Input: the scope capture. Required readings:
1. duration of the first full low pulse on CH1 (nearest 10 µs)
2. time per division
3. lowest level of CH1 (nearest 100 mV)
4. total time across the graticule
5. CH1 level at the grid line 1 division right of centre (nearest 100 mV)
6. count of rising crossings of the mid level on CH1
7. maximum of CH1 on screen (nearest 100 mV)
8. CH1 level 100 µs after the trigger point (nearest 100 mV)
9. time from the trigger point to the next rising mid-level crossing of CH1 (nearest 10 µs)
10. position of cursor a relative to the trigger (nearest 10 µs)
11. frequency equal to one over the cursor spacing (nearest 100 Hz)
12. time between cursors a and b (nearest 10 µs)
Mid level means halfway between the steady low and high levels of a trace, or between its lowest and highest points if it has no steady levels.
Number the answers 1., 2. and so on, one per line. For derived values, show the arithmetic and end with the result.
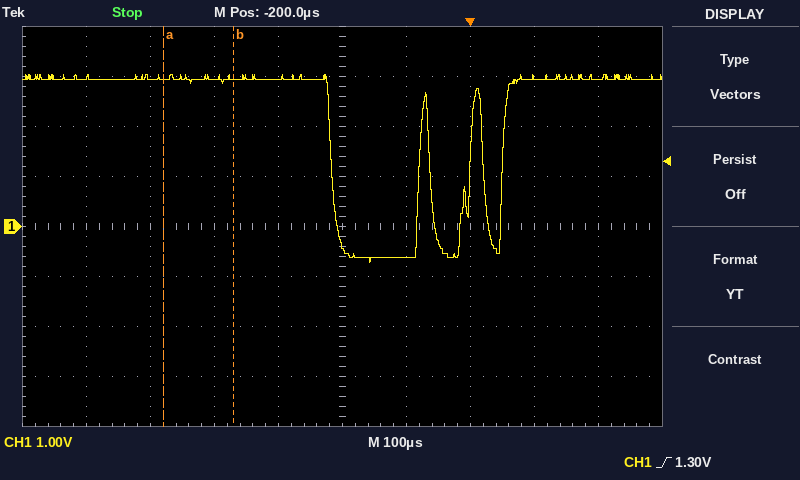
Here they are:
1. 140 µs
2. 100 µs
3. -700 mV
4. 1 ms
5. -600 mV
6. 3
7. 3.0 V
8. 3.0 V
9. 50 µs
10. -480 µs
11. 1 / 110 µs ≈ 9.1 kHz
12. 110 µs
